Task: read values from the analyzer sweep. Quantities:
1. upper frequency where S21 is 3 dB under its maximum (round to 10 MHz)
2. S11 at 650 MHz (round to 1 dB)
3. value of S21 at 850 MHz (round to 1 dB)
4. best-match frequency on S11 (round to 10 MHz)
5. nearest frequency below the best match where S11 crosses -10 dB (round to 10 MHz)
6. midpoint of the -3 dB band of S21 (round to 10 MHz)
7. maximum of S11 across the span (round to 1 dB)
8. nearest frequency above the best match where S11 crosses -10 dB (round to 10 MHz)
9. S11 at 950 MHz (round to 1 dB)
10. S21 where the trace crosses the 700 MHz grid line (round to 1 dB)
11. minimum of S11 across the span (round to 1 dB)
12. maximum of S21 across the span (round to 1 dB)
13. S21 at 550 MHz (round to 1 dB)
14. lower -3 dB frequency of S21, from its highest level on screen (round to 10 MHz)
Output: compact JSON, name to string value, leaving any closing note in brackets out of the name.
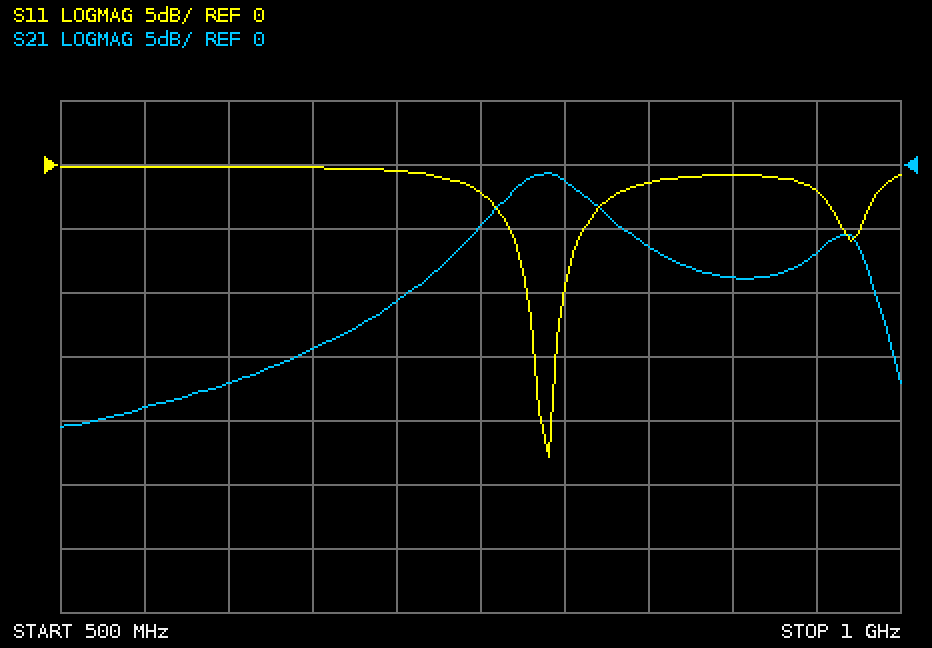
{"upper frequency where S21 is 3 dB under its maximum": "820 MHz", "S11 at 650 MHz": "0 dB", "value of S21 at 850 MHz": "-6 dB", "best-match frequency on S11": "790 MHz", "nearest frequency below the best match where S11 crosses -10 dB": "780 MHz", "midpoint of the -3 dB band of S21": "790 MHz", "maximum of S11 across the span": "0 dB", "nearest frequency above the best match where S11 crosses -10 dB": "800 MHz", "S11 at 950 MHz": "-2 dB", "S21 where the trace crosses the 700 MHz grid line": "-11 dB", "minimum of S11 across the span": "-23 dB", "maximum of S21 across the span": "-1 dB", "S21 at 550 MHz": "-19 dB", "lower -3 dB frequency of S21, from its highest level on screen": "760 MHz"}
